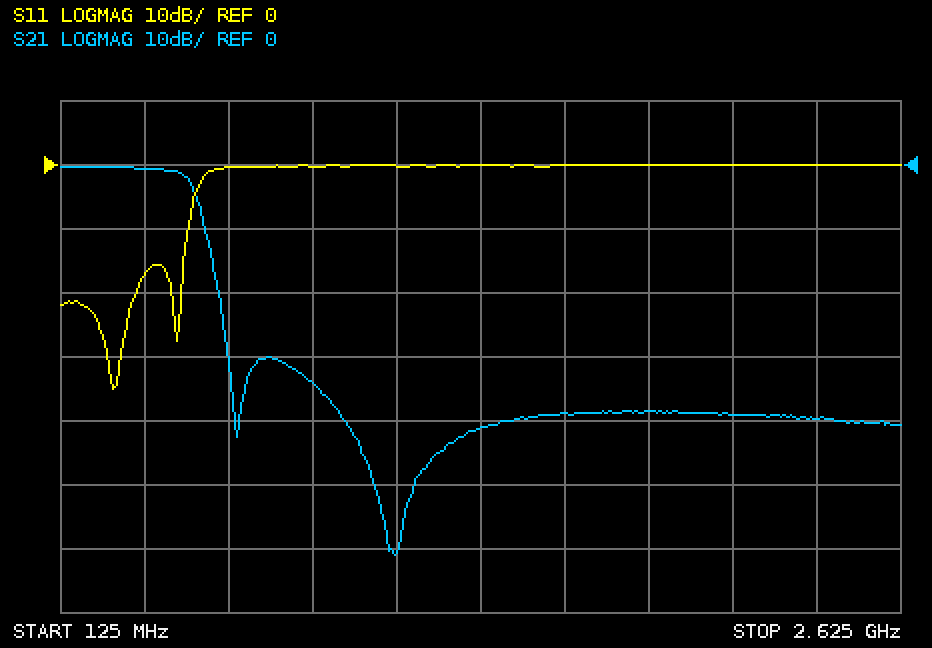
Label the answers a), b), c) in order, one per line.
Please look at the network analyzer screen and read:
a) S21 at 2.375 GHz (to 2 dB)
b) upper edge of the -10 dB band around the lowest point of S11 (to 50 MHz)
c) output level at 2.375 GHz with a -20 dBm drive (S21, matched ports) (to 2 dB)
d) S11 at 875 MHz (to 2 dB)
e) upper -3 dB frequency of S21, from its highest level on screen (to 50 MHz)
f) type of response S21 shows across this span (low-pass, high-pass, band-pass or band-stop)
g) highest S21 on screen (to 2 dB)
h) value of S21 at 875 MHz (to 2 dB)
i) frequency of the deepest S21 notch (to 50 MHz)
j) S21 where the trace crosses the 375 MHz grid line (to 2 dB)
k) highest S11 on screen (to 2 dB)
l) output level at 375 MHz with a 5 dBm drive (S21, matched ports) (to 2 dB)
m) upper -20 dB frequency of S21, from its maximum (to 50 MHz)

a) -40 dB
b) 500 MHz
c) -60 dBm
d) 0 dB
e) 500 MHz
f) low-pass
g) 0 dB
h) -34 dB
i) 1.10 GHz
j) 0 dB
k) 0 dB
l) 4 dBm
m) 600 MHz
